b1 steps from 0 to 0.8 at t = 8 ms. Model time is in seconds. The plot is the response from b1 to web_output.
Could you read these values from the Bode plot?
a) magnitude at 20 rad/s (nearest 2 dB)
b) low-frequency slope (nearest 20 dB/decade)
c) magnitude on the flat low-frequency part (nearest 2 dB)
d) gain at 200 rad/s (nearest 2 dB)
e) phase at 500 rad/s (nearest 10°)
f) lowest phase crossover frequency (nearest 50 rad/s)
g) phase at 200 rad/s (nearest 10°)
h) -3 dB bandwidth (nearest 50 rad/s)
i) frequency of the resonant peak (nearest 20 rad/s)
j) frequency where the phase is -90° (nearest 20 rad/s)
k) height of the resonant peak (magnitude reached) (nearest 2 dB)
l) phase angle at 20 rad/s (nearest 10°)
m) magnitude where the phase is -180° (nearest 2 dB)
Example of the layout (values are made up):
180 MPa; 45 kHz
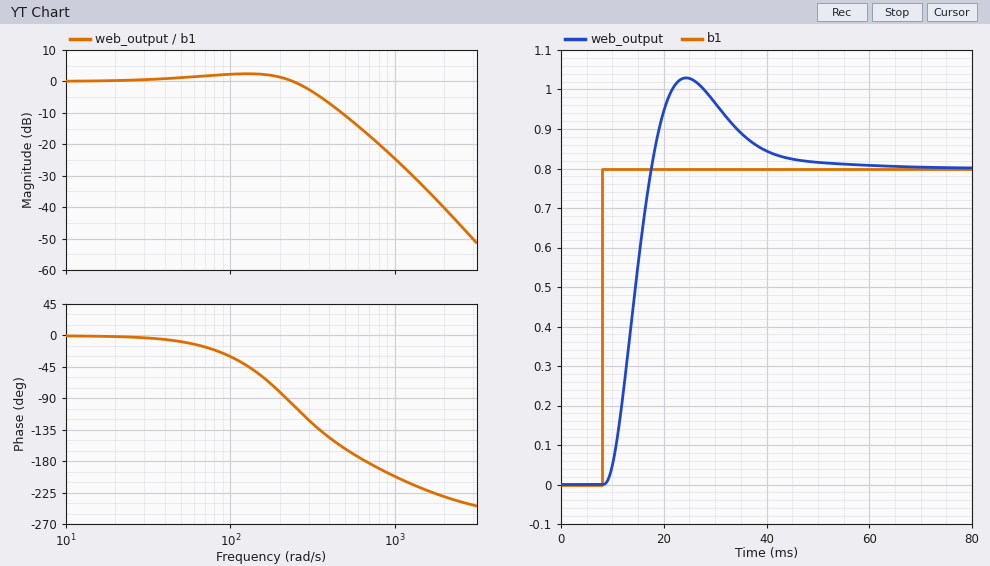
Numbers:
0 dB; 0 dB/decade; 0 dB; 2 dB; -160°; 650 rad/s; -80°; 300 rad/s; 120 rad/s; 220 rad/s; 2 dB; 0°; -16 dB
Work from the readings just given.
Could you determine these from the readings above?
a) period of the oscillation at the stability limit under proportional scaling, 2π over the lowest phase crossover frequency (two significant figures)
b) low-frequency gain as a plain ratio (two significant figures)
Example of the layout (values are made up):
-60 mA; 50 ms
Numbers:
0.0097 s; 1.0
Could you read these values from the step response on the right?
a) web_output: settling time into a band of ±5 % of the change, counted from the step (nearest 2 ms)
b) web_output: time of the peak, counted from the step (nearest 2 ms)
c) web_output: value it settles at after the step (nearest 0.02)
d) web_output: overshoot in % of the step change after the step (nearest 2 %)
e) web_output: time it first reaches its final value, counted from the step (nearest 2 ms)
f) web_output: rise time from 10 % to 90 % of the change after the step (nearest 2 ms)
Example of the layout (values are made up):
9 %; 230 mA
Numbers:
32 ms; 16 ms; 0.80; 28 %; 10 ms; 6 ms
